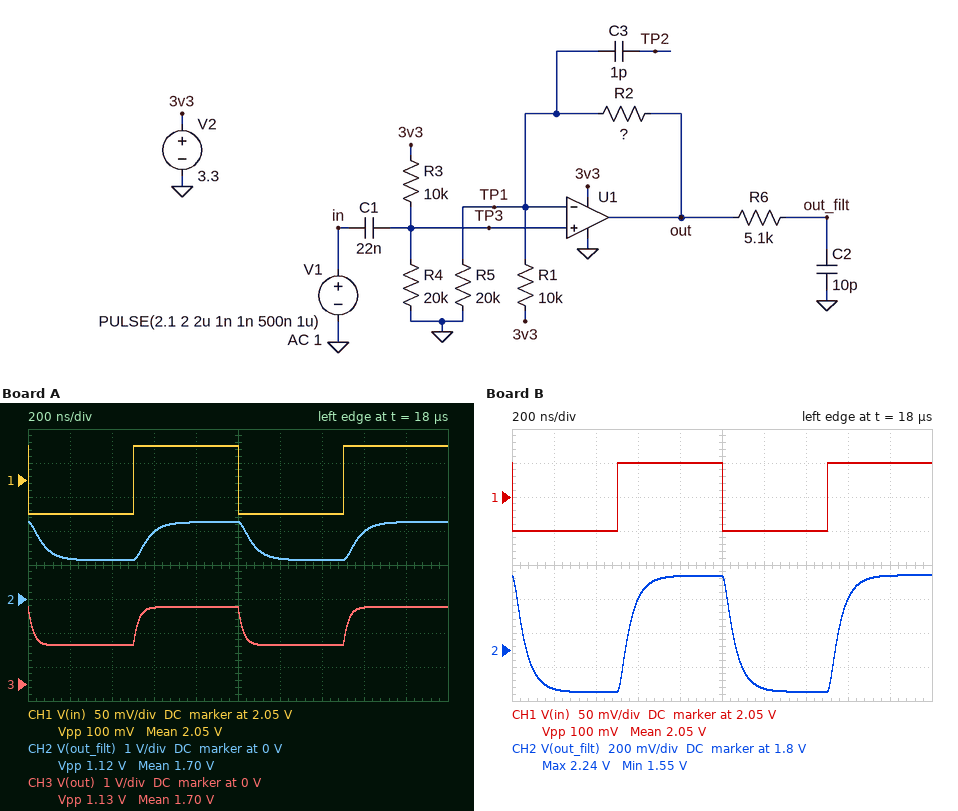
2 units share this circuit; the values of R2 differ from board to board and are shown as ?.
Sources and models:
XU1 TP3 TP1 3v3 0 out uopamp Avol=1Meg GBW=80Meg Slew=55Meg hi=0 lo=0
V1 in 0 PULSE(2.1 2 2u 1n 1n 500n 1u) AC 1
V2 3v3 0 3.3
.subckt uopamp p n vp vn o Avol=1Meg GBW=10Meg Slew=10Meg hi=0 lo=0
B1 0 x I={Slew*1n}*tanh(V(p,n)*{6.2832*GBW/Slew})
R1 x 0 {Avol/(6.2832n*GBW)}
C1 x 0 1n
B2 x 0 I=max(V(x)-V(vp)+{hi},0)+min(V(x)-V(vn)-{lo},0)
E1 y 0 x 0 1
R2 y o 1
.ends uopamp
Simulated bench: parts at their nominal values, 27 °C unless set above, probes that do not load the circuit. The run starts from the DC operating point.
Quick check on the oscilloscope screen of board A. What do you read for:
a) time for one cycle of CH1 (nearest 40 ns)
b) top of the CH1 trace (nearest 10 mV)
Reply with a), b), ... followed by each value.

a) 1.00 µs
b) 2.10 V
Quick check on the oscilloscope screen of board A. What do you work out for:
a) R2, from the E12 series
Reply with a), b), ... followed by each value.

a) 68 kΩ
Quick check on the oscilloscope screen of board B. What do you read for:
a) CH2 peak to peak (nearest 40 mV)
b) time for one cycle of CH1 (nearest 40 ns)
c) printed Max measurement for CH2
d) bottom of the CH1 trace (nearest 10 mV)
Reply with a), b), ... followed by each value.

a) 680 mV
b) 1.00 µs
c) 2.24 V
d) 2.00 V
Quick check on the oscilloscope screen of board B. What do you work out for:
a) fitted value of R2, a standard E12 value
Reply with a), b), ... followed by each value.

a) 39 kΩ
